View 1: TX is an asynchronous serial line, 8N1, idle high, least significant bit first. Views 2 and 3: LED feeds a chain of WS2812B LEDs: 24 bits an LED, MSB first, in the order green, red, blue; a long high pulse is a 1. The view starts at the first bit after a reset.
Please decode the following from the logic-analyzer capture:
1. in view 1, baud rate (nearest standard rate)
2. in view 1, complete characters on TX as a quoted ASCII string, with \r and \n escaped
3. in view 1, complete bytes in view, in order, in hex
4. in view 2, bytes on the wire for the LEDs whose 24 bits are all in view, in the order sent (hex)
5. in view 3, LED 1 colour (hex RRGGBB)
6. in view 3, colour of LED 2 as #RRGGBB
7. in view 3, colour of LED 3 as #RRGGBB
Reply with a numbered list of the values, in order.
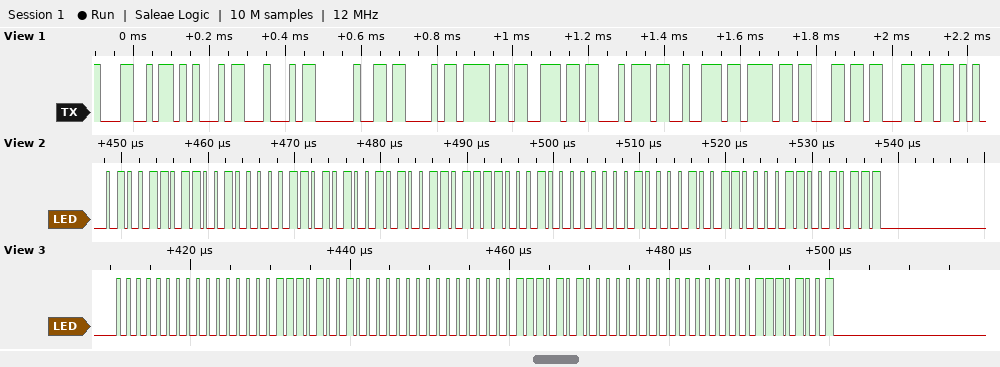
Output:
1. 57600 baud
2. "LED Controll"
3. 4C 45 44 20 43 6F 6E 74 72 6F 6C 6C
4. 4D 90 6A 53 78 80 42 61 97
5. #0000E9
6. #0000EA
7. #0000E9
